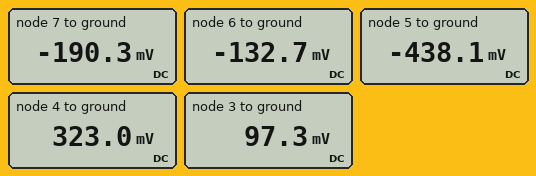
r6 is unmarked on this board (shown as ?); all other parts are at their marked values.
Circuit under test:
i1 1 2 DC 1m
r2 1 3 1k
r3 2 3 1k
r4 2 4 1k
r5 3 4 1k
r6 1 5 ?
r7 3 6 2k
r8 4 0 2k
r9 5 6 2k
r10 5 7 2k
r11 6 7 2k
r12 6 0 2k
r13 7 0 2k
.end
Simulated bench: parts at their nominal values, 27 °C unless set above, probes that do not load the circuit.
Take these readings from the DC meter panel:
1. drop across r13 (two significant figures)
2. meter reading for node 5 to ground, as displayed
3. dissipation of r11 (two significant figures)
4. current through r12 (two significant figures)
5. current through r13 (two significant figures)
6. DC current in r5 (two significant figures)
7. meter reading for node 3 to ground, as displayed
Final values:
190 mV
-438.1 mV
1.7 µW
66 µA
95 µA
230 µA
97.3 mV
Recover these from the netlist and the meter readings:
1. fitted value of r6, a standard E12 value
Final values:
680 Ω
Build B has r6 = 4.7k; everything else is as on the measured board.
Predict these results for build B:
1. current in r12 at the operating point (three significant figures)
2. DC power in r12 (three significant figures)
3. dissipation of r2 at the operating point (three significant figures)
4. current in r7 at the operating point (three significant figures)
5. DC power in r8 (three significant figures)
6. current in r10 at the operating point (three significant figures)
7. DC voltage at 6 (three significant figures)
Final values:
50.9 µA
5.18 µW
741 µW
29.9 µA
23.9 µW
65.9 µA
-102 mV
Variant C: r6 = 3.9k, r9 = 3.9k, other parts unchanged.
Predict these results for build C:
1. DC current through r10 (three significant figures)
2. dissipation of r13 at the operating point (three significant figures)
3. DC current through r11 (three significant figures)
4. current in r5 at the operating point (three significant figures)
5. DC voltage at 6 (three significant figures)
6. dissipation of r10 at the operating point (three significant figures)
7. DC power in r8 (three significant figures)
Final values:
89.2 µA
9.19 µW
21.4 µA
257 µA
-92.7 mV
15.9 µW
26.0 µW
